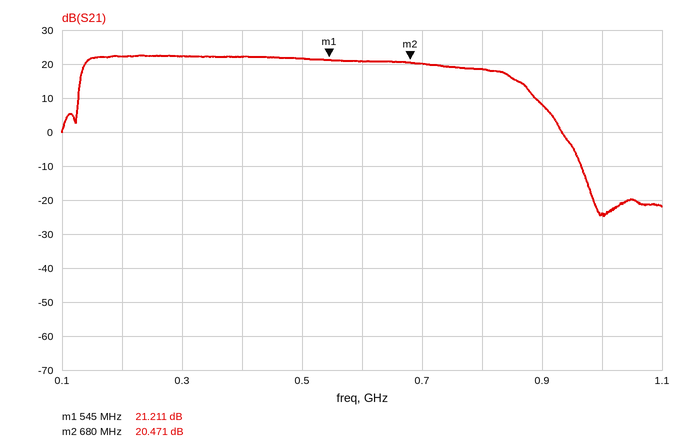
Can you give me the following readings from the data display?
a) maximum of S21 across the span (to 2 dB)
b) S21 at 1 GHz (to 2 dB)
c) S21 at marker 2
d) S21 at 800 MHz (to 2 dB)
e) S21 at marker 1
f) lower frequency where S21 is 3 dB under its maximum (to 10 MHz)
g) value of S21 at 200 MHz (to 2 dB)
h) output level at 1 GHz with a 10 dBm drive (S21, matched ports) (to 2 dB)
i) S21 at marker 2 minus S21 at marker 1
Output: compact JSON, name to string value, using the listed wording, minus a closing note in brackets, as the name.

{"maximum of S21 across the span": "22 dB", "S21 at 1 GHz": "-24 dB", "S21 at marker 2": "20.471 dB", "S21 at 800 MHz": "18 dB", "S21 at marker 1": "21.211 dB", "lower frequency where S21 is 3 dB under its maximum": "140 MHz", "value of S21 at 200 MHz": "22 dB", "output level at 1 GHz with a 10 dBm drive (S21, matched ports)": "-14 dBm", "S21 at marker 2 minus S21 at marker 1": "-0.740 dB"}
